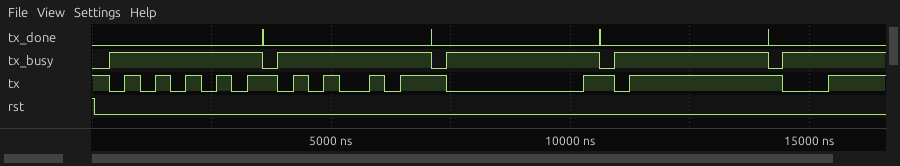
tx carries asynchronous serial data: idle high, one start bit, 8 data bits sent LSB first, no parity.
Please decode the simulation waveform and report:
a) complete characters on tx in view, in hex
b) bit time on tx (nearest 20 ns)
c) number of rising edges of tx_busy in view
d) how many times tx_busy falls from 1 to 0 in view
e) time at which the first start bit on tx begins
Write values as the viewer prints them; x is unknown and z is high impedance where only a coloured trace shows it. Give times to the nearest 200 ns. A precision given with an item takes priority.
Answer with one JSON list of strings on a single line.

["55, A5, 00, FF", "320 ns", "5", "4", "400 ns"]
